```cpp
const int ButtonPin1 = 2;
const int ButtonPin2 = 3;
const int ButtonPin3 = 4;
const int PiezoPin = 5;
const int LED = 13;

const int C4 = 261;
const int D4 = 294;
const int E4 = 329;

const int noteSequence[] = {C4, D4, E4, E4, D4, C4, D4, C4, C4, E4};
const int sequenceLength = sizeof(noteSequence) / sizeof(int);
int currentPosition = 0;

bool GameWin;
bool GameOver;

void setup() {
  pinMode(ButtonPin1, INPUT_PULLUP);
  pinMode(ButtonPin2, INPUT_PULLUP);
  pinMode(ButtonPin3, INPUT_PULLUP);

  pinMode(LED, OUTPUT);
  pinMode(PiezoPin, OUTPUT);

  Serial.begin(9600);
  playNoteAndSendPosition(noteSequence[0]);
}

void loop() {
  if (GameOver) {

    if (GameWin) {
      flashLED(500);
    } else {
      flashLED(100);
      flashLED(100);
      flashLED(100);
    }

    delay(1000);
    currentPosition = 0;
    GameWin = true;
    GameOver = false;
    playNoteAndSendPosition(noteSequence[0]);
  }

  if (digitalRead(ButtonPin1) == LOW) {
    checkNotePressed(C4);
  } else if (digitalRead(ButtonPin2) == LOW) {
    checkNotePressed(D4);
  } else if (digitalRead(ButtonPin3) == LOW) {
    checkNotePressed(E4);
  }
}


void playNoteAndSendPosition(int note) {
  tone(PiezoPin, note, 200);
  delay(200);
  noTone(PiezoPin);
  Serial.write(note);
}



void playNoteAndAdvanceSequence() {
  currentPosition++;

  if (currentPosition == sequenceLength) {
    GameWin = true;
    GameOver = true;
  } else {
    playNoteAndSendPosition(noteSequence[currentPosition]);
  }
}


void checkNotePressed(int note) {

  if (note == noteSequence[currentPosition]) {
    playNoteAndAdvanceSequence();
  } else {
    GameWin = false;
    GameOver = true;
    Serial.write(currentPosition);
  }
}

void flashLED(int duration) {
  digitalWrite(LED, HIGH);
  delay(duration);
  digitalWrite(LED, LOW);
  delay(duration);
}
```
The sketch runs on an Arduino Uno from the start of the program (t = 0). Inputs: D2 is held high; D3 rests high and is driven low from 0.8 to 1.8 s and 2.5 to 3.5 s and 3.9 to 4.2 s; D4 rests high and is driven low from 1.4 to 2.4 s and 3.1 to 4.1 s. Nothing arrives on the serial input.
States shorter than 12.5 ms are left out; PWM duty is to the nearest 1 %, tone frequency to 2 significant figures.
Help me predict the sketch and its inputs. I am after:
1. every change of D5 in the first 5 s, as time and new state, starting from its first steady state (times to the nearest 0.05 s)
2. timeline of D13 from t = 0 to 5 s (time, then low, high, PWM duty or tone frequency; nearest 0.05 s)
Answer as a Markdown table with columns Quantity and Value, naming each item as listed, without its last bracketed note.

| Quantity | Value |
|---|---|
| every change of D5 in the first 5 s, as time and new state, starting from its first steady state | 0 s tone 260 Hz; 0.2 s low; 2.4 s tone 260 Hz; 2.6 s low; 4.2 s tone 260 Hz; 4.4 s low |
| timeline of D13 from t = 0 to 5 s | 0 s low; 0.8 s high; 0.9 s low; 1 s high; 1.1 s low; 1.2 s high; 1.3 s low; 2.6 s high; 2.7 s low; 2.8 s high; 2.9 s low; 3 s high; 3.1 s low |
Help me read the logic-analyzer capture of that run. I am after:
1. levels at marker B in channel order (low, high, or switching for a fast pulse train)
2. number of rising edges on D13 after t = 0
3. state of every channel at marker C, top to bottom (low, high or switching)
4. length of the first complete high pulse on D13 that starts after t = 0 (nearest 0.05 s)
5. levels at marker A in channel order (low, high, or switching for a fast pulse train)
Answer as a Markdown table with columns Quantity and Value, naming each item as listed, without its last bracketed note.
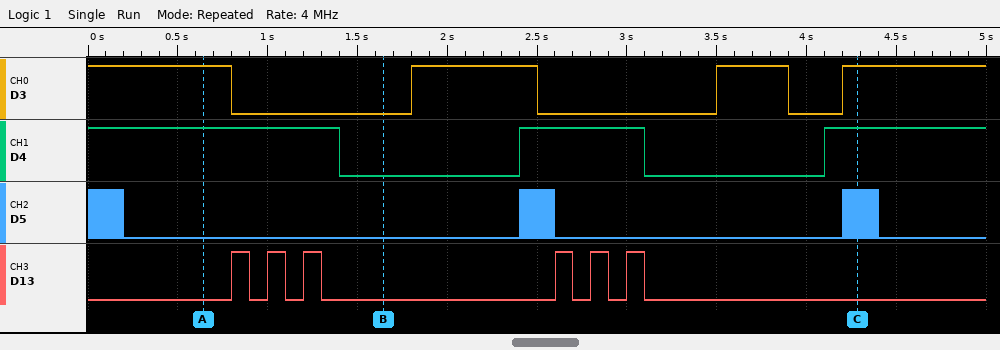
| Quantity | Value |
|---|---|
| levels at marker B in channel order | D3 low, D4 low, D5 low, D13 low |
| number of rising edges on D13 after t = 0 | 6 |
| state of every channel at marker C, top to bottom | D3 high, D4 high, D5 switching, D13 low |
| length of the first complete high pulse on D13 that starts after t = 0 | 0.10 s |
| levels at marker A in channel order | D3 high, D4 high, D5 low, D13 low |
